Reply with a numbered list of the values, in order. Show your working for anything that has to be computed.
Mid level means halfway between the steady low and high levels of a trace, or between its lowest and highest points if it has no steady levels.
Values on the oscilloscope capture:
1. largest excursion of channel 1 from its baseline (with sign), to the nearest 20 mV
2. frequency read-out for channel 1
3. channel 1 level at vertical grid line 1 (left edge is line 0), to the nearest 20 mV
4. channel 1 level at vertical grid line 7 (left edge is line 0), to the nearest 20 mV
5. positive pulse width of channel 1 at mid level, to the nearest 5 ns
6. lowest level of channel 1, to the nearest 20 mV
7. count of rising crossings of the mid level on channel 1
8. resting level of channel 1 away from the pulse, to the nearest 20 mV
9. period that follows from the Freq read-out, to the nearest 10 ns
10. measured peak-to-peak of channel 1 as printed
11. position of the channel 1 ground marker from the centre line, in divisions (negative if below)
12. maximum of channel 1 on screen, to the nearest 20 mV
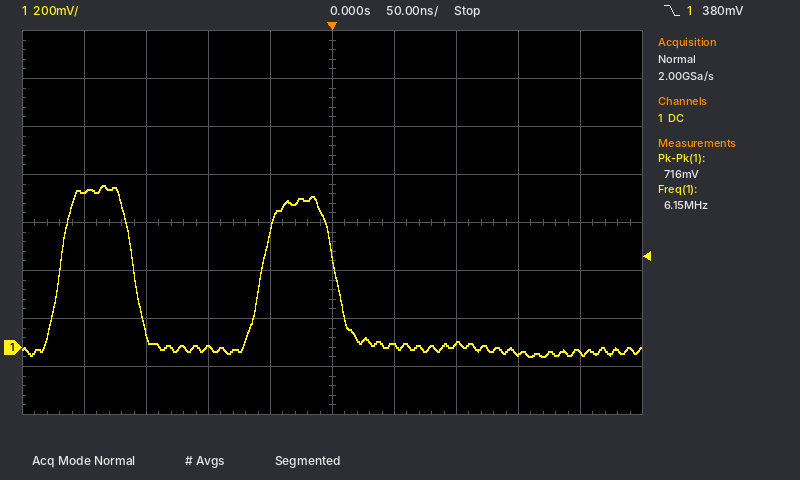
1. 680 mV − (0 mV) = +680 mV
2. 6.15 MHz
3. 640 mV
4. 20 mV
5. 60 ns
6. -40 mV
7. 2
8. 0 mV
9. 1 / 6.15 MHz ≈ 163 ns, so 160 ns to the nearest 10 ns
10. 716 mV
11. -2.6 div
12. 680 mV
